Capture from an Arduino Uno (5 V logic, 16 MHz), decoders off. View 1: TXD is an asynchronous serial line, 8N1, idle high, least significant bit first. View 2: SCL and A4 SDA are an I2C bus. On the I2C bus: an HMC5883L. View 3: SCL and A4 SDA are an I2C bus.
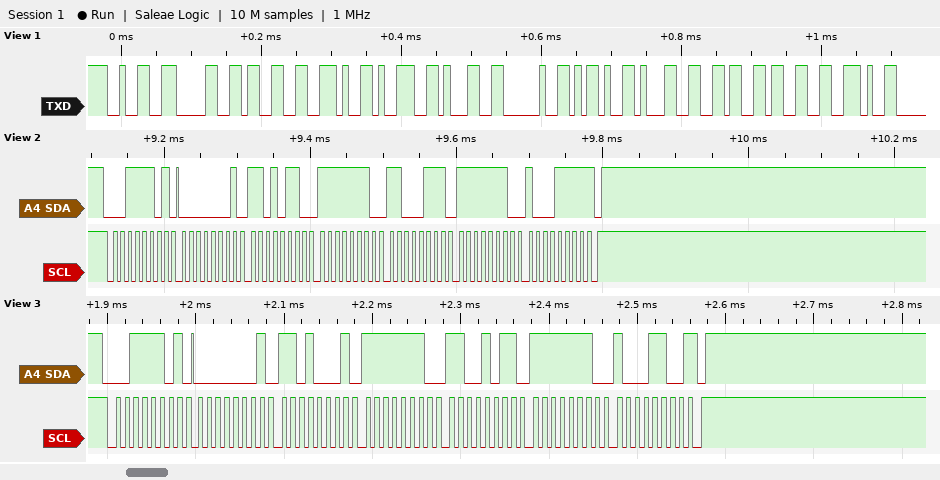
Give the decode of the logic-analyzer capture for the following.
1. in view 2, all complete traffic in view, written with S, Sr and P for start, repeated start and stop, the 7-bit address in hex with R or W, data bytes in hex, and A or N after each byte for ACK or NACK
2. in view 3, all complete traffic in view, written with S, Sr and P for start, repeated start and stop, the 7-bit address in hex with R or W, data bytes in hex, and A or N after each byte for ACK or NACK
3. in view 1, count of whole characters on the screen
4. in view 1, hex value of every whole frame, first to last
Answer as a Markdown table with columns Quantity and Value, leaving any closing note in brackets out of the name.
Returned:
| Quantity | Value |
|---|---|
| in view 2, all complete traffic in view, written with S, Sr and P for start, repeated start and stop, the 7-bit address in hex with R or W, data bytes in hex, and A or N after each byte for ACK or NACK | S 1ER A 01 A D6 A FE A C7 A FE A 8F N P |
| in view 3, all complete traffic in view, written with S, Sr and P for start, repeated start and stop, the 7-bit address in hex with R or W, data bytes in hex, and A or N after each byte for ACK or NACK | S 1ER A 01 A D1 A FE A CB A FE A 8C N P |
| in view 1, count of whole characters on the screen | 12 |
| in view 1, hex value of every whole frame, first to last | 32 30 33 2E 39 31 20 2D 31 36 33 2E |
